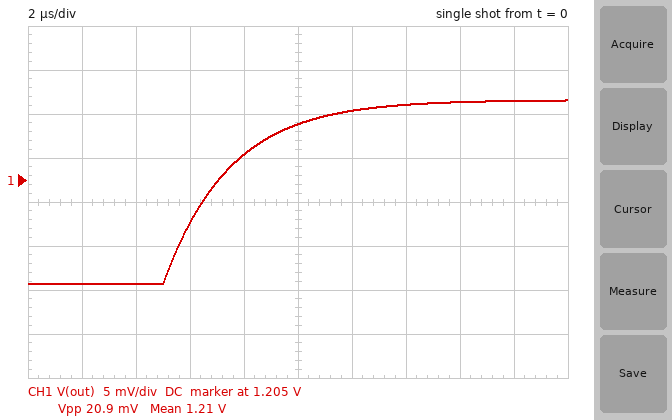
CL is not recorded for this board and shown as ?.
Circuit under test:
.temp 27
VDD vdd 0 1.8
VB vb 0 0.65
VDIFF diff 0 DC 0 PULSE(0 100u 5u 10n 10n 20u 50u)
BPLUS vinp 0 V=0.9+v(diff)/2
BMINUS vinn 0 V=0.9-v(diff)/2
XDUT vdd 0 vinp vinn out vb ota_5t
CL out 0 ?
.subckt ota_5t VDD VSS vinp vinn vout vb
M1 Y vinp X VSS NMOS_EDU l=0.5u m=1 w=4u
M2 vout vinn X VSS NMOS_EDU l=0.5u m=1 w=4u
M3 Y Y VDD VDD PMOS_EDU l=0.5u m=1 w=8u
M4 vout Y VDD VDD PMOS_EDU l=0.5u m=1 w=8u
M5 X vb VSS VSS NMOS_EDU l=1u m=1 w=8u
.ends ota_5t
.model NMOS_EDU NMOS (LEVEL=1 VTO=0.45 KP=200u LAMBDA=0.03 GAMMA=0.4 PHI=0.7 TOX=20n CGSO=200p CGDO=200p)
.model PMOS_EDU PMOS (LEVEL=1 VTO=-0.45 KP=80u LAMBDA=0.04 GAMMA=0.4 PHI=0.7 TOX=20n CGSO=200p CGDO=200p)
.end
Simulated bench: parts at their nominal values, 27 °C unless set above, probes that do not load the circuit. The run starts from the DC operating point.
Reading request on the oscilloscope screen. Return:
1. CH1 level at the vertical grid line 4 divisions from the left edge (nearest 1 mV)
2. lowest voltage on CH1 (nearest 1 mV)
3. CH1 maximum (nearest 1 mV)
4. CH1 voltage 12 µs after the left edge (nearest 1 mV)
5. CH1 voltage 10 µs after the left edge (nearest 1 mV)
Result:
1.208 V
1.193 V
1.214 V
1.213 V
1.211 V
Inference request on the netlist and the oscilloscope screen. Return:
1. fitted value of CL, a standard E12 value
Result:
2.7 pF
